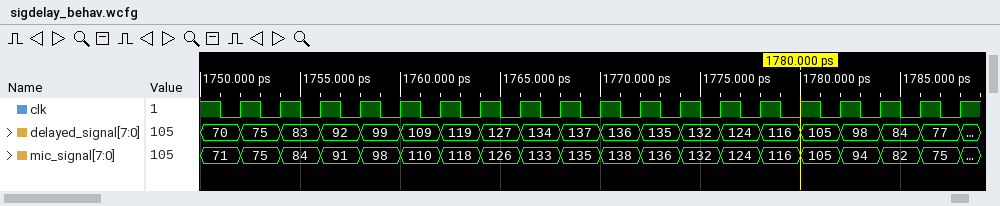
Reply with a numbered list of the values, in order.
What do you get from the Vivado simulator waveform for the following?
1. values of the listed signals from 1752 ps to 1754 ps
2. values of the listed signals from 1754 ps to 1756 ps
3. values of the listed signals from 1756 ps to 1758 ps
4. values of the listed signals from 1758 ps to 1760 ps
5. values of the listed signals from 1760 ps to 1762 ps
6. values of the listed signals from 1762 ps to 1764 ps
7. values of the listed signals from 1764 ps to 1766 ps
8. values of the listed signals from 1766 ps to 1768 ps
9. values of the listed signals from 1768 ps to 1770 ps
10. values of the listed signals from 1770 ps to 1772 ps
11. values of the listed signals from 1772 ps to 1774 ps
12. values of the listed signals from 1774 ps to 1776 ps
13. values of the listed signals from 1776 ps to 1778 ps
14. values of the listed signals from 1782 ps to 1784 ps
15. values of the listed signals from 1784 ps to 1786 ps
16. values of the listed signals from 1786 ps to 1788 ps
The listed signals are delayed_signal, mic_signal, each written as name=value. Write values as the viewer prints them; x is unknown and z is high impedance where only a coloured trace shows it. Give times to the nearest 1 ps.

1. delayed_signal=75, mic_signal=75
2. delayed_signal=83, mic_signal=84
3. delayed_signal=92, mic_signal=91
4. delayed_signal=99, mic_signal=98
5. delayed_signal=109, mic_signal=110
6. delayed_signal=119, mic_signal=118
7. delayed_signal=127, mic_signal=126
8. delayed_signal=134, mic_signal=133
9. delayed_signal=137, mic_signal=135
10. delayed_signal=136, mic_signal=138
11. delayed_signal=135, mic_signal=136
12. delayed_signal=132, mic_signal=132
13. delayed_signal=124, mic_signal=124
14. delayed_signal=98, mic_signal=94
15. delayed_signal=84, mic_signal=82
16. delayed_signal=77, mic_signal=75
